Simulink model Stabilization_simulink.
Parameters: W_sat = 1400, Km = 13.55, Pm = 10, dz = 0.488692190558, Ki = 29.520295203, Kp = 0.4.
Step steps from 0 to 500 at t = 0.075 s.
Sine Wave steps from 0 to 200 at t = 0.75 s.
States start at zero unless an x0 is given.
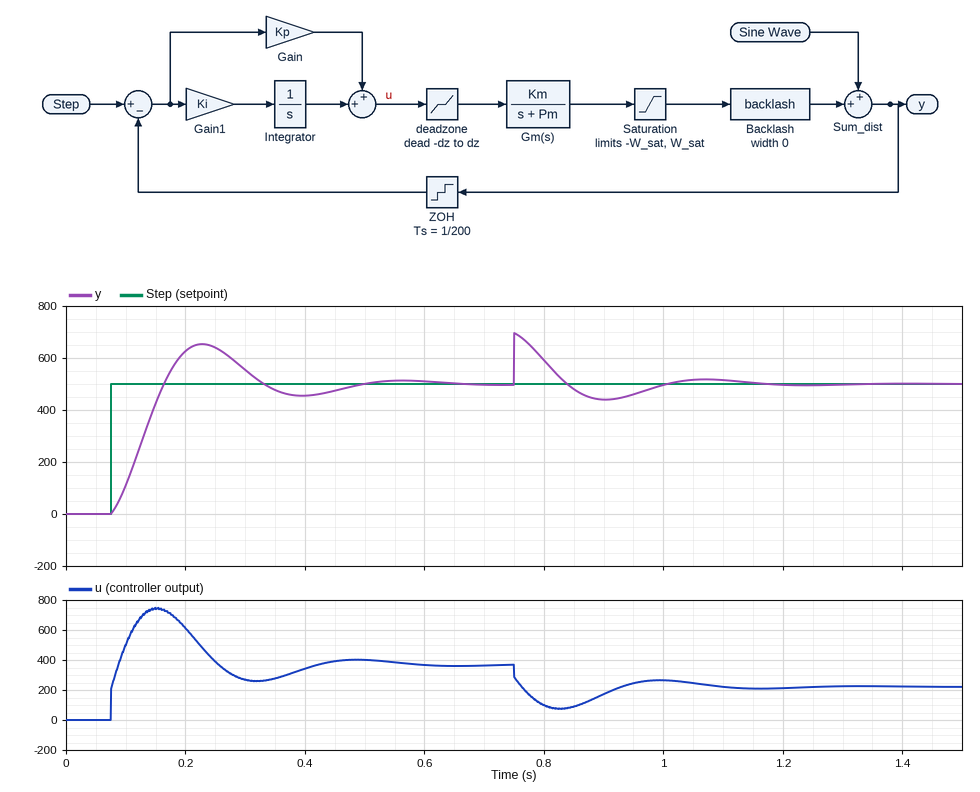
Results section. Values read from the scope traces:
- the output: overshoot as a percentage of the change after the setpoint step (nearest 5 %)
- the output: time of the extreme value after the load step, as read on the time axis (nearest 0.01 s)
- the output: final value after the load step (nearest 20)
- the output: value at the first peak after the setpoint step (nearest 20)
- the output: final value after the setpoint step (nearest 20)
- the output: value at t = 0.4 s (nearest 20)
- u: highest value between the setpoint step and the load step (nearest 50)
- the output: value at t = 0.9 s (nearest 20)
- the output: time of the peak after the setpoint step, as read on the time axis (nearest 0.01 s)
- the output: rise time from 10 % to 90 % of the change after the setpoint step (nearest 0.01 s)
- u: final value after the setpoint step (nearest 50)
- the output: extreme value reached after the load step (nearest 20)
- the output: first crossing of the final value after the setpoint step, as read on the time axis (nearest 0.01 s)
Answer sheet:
30 %
0.75 s
500
660
500
460
750
440
0.23 s
0.07 s
350
700
0.16 s
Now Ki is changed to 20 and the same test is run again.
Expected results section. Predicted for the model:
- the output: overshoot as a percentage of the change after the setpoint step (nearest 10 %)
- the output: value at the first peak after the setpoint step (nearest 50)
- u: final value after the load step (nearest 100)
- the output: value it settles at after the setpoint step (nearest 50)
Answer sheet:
20 %
600
200
500
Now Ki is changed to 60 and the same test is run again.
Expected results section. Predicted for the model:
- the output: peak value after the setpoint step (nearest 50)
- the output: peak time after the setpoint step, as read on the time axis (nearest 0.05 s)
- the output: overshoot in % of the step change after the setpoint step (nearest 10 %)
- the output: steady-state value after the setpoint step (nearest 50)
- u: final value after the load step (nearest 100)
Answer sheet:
750
0.20 s
50 %
500
200
